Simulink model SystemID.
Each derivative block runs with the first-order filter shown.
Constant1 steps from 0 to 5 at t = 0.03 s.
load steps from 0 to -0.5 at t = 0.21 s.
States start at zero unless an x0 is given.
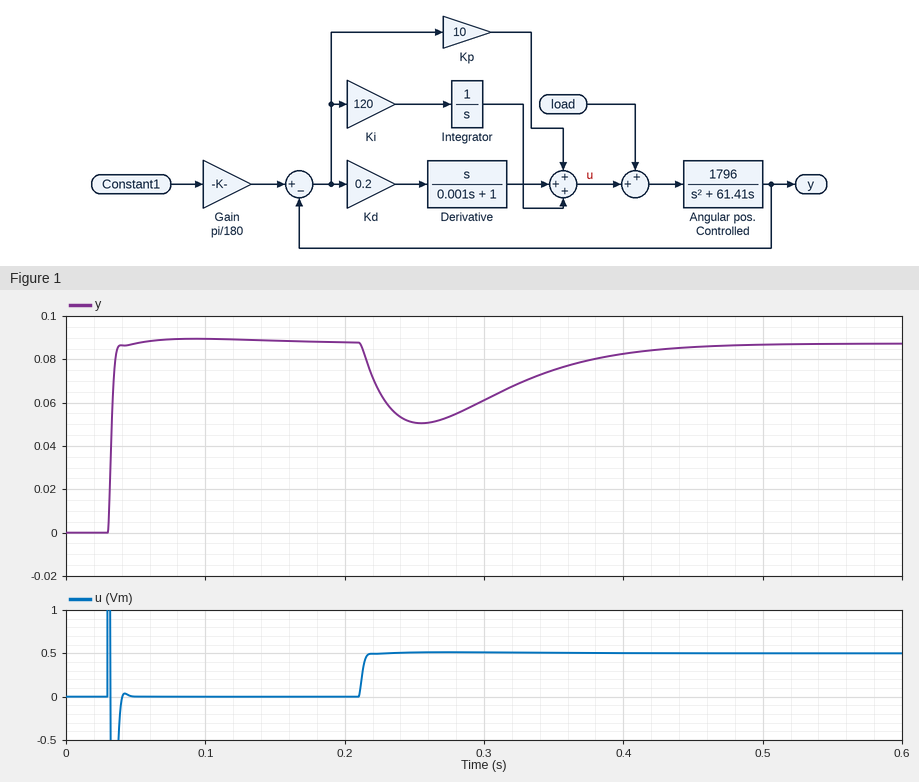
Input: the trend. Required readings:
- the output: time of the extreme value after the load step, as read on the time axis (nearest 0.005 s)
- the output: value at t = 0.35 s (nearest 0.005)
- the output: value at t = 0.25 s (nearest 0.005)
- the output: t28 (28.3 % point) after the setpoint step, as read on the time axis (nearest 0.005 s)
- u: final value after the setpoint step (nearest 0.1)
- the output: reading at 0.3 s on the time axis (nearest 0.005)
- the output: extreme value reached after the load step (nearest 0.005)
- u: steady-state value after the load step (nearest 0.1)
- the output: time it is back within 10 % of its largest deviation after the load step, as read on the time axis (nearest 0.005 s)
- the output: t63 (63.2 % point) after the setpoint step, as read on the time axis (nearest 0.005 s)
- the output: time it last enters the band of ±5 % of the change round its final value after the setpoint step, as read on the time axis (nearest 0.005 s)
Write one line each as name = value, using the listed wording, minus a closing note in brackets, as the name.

the output: time of the extreme value after the load step, as read on the time axis = 0.255 s
the output: value at t = 0.35 s = 0.075
the output: value at t = 0.25 s = 0.050
the output: t28 (28.3 % point) after the setpoint step, as read on the time axis = 0.030 s
u: final value after the setpoint step = 0.0
the output: reading at 0.3 s on the time axis = 0.060
the output: extreme value reached after the load step = 0.050
u: steady-state value after the load step = 0.5
the output: time it is back within 10 % of its largest deviation after the load step, as read on the time axis = 0.410 s
the output: t63 (63.2 % point) after the setpoint step, as read on the time axis = 0.035 s
the output: time it last enters the band of ±5 % of the change round its final value after the setpoint step, as read on the time axis = 0.035 s
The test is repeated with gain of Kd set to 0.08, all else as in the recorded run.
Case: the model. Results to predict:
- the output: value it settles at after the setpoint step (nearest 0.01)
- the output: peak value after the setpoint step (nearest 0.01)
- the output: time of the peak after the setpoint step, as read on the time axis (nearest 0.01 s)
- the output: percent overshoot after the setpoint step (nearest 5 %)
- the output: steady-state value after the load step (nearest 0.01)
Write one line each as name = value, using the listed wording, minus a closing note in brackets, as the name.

the output: value it settles at after the setpoint step = 0.09
the output: peak value after the setpoint step = 0.10
the output: time of the peak after the setpoint step, as read on the time axis = 0.05 s
the output: percent overshoot after the setpoint step = 15 %
the output: steady-state value after the load step = 0.09
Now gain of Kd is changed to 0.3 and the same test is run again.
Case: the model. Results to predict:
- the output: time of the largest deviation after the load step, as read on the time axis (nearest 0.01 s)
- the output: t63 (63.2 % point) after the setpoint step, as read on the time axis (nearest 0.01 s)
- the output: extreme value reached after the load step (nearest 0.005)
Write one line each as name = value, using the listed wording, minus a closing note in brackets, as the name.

the output: time of the largest deviation after the load step, as read on the time axis = 0.27 s
the output: t63 (63.2 % point) after the setpoint step, as read on the time axis = 0.03 s
the output: extreme value reached after the load step = 0.055
